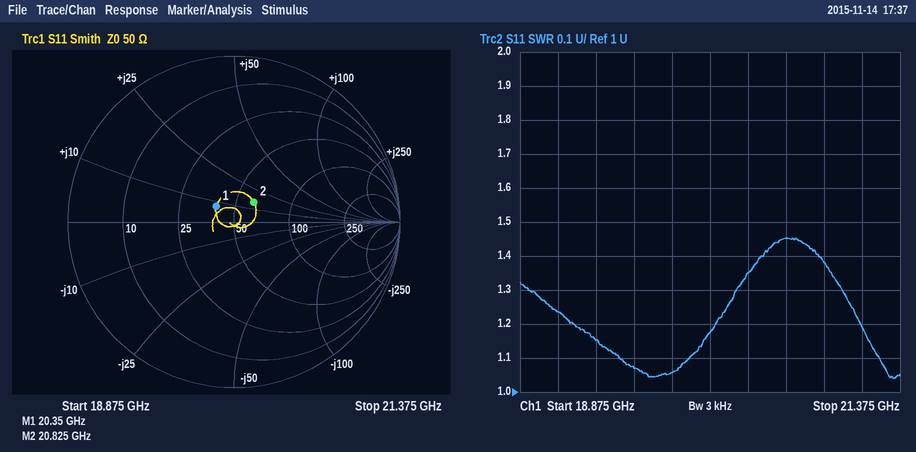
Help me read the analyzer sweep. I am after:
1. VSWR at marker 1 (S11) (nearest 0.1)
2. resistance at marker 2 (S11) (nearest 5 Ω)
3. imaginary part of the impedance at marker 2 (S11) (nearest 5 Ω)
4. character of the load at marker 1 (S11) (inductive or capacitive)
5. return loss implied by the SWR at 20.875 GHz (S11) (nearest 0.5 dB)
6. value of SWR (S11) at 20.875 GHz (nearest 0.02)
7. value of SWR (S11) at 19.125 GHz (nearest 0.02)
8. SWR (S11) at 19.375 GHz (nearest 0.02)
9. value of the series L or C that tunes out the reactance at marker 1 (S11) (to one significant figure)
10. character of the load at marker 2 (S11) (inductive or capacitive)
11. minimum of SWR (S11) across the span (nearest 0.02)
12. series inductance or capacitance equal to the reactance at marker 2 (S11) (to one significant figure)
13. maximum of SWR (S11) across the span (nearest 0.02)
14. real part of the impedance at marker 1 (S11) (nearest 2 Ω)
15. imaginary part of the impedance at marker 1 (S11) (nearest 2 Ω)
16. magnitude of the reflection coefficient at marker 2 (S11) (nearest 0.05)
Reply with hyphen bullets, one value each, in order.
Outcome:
- 1.3
- 60 Ω
- +15 Ω
- inductive
- 16.0 dB
- 1.38
- 1.24
- 1.16
- 1 pF
- inductive
- 1.04
- 100 pH
- 1.46
- 40 Ω
- +8 Ω
- 0.15
